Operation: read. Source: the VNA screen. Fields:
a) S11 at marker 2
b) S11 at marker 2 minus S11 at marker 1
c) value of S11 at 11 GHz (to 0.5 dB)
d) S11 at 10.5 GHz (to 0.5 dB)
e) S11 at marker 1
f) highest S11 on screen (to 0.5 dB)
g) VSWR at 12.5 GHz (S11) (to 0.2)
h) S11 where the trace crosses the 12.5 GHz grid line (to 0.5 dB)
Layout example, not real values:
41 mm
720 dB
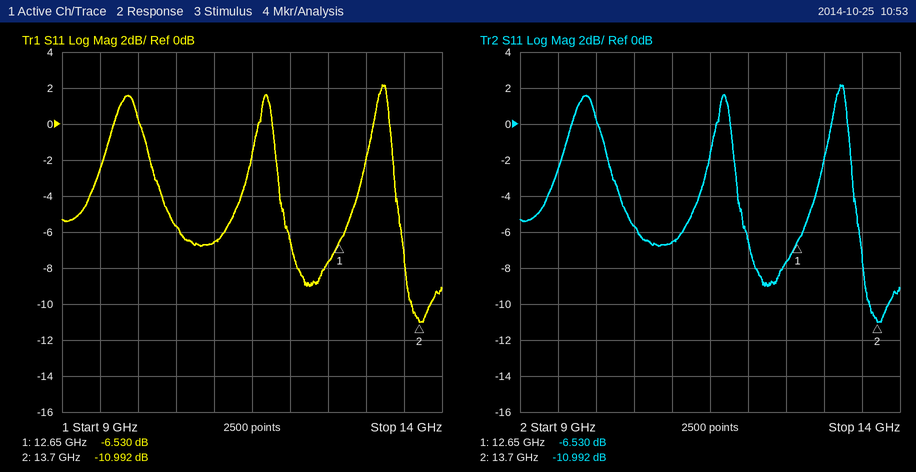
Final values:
-10.992 dB
-4.462 dB
-6.5 dB
-5.5 dB
-6.530 dB
2.0 dB
2.4
-7.5 dB
